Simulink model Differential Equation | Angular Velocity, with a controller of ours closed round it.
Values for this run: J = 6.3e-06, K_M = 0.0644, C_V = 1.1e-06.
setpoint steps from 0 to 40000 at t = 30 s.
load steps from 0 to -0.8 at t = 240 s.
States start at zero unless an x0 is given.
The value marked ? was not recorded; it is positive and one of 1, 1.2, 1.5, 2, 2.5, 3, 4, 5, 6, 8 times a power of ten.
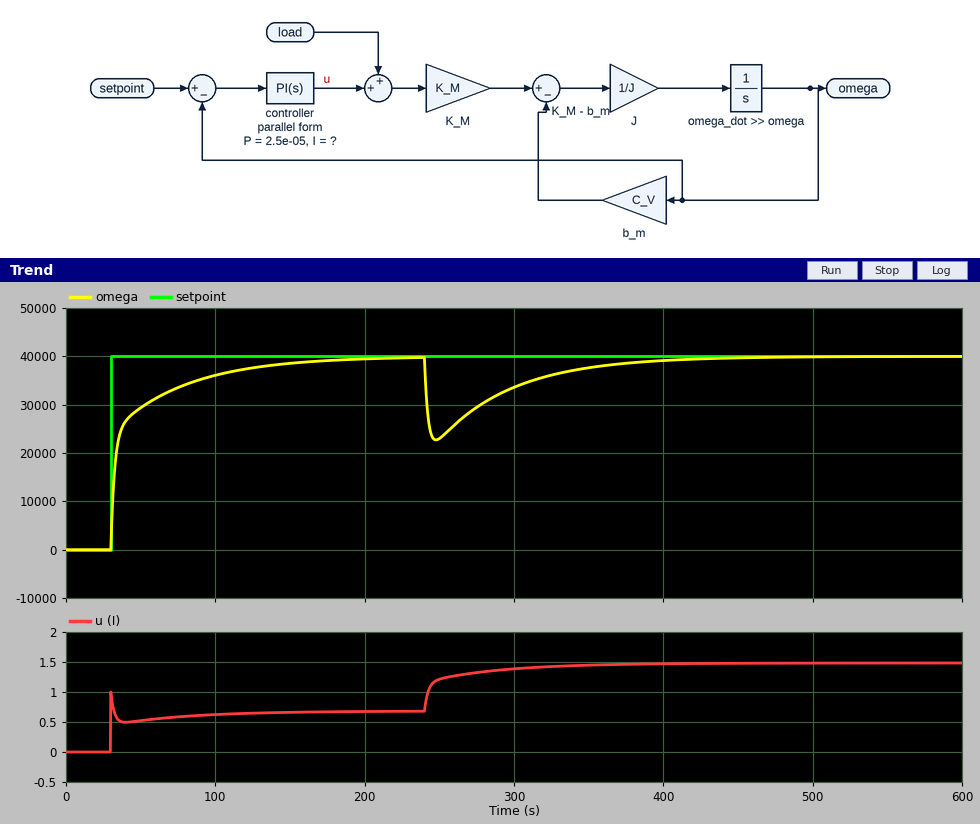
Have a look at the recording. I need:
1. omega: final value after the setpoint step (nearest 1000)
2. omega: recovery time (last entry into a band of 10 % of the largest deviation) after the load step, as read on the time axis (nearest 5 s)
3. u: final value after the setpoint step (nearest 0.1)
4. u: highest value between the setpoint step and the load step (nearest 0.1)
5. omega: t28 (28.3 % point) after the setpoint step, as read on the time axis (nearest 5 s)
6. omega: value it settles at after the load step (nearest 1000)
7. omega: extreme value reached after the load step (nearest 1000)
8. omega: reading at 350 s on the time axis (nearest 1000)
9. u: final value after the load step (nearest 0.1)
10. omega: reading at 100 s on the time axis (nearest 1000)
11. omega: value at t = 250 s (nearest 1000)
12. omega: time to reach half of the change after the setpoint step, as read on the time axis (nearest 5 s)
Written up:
40000
365 s
0.7
1.0
30 s
40000
23000
38000
1.5
36000
23000
35 s
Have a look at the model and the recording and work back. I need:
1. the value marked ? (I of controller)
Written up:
8e-07
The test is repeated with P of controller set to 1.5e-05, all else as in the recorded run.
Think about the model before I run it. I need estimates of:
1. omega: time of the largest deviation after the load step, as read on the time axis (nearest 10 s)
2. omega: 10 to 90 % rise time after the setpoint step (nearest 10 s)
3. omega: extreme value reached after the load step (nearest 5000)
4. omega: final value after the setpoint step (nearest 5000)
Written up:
250 s
60 s
20000
40000
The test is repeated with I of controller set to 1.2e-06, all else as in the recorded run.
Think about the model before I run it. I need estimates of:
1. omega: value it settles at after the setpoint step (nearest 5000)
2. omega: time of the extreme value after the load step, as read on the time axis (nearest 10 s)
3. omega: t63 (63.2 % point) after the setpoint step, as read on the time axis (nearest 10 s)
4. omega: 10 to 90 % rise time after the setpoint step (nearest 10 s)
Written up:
40000
250 s
40 s
40 s
